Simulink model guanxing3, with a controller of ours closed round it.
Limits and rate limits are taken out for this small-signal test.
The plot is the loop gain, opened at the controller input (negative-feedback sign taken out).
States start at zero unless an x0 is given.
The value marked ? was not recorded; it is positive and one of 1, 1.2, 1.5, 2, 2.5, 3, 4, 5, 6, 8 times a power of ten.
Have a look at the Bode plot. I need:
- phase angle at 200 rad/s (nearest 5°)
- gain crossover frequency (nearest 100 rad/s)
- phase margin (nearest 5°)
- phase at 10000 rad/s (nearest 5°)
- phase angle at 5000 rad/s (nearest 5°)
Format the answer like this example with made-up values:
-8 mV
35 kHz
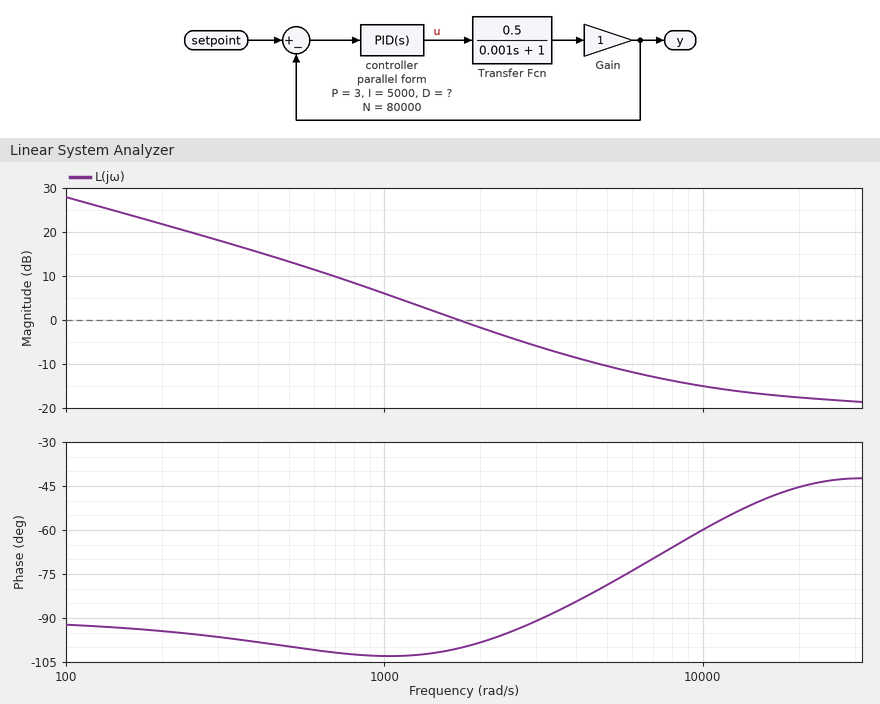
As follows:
-95°
1700 rad/s
80°
-60°
-80°
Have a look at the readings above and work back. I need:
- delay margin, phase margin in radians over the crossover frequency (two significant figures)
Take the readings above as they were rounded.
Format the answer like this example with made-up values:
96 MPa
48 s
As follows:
0.00082 s
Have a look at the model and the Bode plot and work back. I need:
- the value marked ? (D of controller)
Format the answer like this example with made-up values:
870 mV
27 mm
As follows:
0.0002
